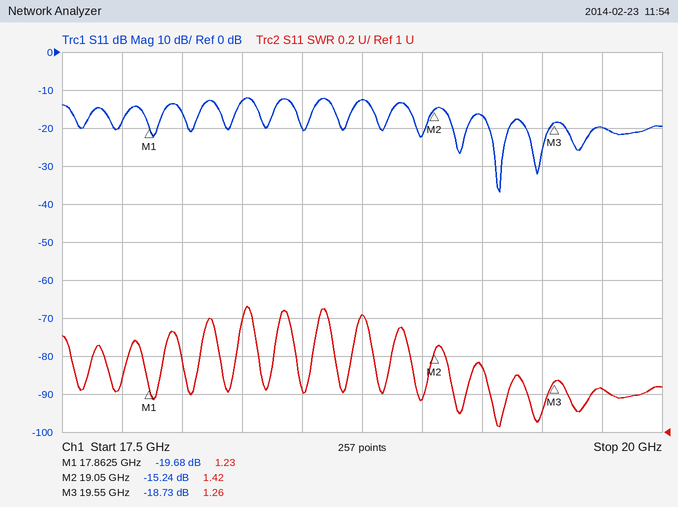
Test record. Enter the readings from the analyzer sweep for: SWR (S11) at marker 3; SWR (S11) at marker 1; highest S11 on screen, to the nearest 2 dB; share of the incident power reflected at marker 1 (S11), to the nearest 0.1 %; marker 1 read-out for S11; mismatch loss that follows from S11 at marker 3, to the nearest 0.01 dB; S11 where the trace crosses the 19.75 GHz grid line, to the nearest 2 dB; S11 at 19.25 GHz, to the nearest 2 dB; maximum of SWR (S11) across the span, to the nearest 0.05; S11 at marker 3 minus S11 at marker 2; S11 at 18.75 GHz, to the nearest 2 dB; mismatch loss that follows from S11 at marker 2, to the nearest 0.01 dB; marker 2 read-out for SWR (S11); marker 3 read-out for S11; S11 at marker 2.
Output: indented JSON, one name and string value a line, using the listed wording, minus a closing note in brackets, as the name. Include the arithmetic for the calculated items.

{
  "SWR (S11) at marker 3": "1.26",
  "SWR (S11) at marker 1": "1.23",
  "highest S11 on screen, to the nearest 2 dB": "-12 dB",
  "share of the incident power reflected at marker 1 (S11), to the nearest 0.1 %": "10^(-19.68/10) ≈ 1.1 %",
  "marker 1 read-out for S11": "-19.68 dB",
  "mismatch loss that follows from S11 at marker 3, to the nearest 0.01 dB": "−10 log10(1 − 10^(-18.73/10)) ≈ 0.06 dB",
  "S11 where the trace crosses the 19.75 GHz grid line, to the nearest 2 dB": "-20 dB",
  "S11 at 19.25 GHz, to the nearest 2 dB": "-16 dB",
  "maximum of SWR (S11) across the span, to the nearest 0.05": "1.65",
  "S11 at marker 3 minus S11 at marker 2": "-18.73 − (-15.24) = -3.49 dB",
  "S11 at 18.75 GHz, to the nearest 2 dB": "-12 dB",
  "mismatch loss that follows from S11 at marker 2, to the nearest 0.01 dB": "−10 log10(1 − 10^(-15.24/10)) ≈ 0.13 dB",
  "marker 2 read-out for SWR": "1.42",
  "marker 3 read-out for S11": "-18.73 dB",
  "S11 at marker 2": "-15.24 dB"
}
